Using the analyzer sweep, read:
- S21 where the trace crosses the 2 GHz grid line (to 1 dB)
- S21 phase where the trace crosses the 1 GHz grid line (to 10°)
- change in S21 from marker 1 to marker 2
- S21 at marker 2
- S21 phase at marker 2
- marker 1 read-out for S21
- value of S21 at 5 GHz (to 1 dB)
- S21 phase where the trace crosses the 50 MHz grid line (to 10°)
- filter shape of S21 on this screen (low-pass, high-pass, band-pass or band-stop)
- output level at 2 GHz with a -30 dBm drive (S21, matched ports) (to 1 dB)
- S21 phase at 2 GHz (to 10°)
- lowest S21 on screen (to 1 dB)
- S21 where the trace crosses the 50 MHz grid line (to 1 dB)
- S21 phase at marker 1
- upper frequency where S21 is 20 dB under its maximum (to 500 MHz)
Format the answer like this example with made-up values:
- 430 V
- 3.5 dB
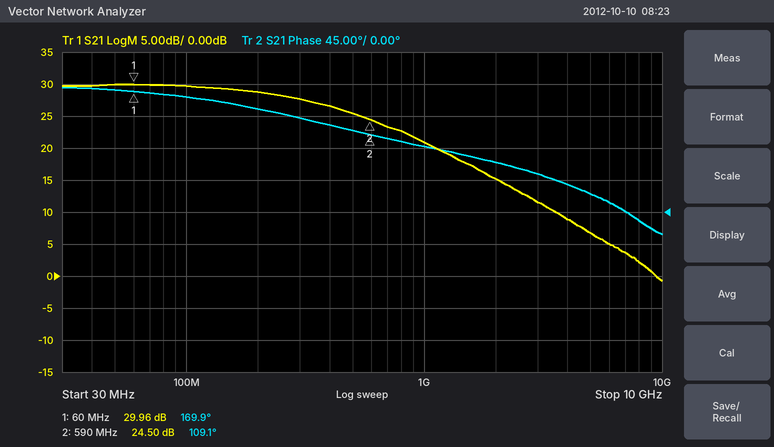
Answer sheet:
- 15 dB
- 90°
- -5.46 dB
- 24.50 dB
- 109.1°
- 29.96 dB
- 7 dB
- 170°
- low-pass
- -15 dBm
- 70°
- -1 dB
- 30 dB
- 169.9°
- 3.5 GHz
